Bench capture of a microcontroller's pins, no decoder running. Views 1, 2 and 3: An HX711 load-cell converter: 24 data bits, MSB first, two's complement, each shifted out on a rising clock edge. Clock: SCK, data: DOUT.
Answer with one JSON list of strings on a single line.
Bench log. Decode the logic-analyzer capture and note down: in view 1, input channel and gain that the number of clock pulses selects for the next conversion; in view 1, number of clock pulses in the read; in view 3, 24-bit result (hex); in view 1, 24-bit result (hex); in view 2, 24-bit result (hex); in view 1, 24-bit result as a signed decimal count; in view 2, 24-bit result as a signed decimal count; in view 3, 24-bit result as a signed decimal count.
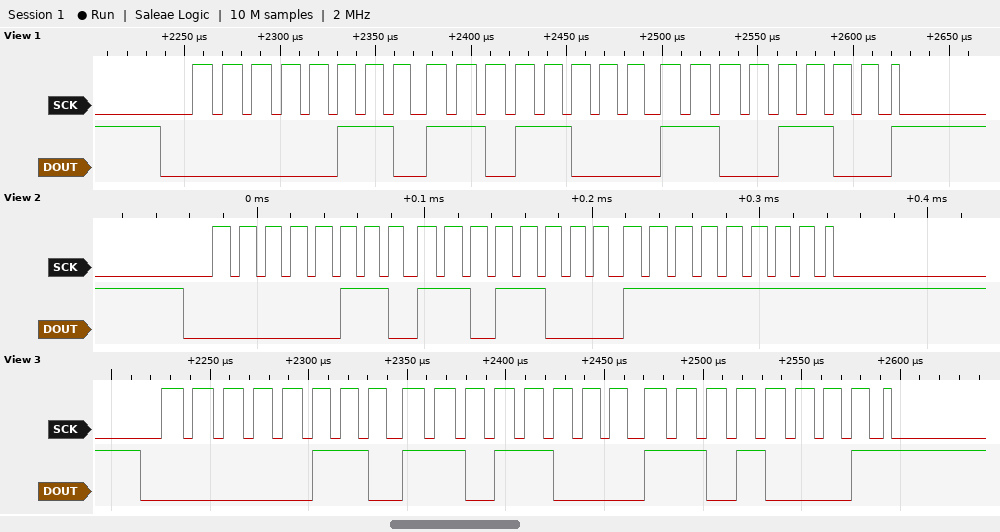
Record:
["channel A, gain 128", "25", "0x06D8D1", "0x06D8CC", "0x06D8FF", "448716", "448767", "448721"]
